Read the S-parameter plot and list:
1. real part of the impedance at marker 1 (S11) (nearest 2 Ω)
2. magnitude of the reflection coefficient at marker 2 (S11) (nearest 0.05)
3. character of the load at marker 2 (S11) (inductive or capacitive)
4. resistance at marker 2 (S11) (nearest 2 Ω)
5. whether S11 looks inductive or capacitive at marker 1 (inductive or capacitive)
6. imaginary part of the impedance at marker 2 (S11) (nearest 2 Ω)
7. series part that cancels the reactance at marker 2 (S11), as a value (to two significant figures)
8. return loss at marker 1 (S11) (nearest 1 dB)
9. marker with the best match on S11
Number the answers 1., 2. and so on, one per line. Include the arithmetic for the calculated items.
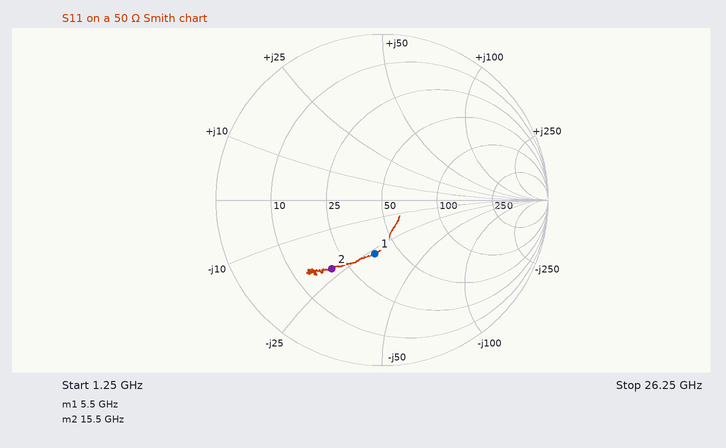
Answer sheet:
1. 38 Ω
2. 0.50
3. capacitive
4. 20 Ω
5. capacitive
6. -22 Ω
7. L = 22 Ω/(2π × 15.5 GHz) ≈ 226 pH, so 230 pH to two significant figures
8. 10 dB
9. marker 1
